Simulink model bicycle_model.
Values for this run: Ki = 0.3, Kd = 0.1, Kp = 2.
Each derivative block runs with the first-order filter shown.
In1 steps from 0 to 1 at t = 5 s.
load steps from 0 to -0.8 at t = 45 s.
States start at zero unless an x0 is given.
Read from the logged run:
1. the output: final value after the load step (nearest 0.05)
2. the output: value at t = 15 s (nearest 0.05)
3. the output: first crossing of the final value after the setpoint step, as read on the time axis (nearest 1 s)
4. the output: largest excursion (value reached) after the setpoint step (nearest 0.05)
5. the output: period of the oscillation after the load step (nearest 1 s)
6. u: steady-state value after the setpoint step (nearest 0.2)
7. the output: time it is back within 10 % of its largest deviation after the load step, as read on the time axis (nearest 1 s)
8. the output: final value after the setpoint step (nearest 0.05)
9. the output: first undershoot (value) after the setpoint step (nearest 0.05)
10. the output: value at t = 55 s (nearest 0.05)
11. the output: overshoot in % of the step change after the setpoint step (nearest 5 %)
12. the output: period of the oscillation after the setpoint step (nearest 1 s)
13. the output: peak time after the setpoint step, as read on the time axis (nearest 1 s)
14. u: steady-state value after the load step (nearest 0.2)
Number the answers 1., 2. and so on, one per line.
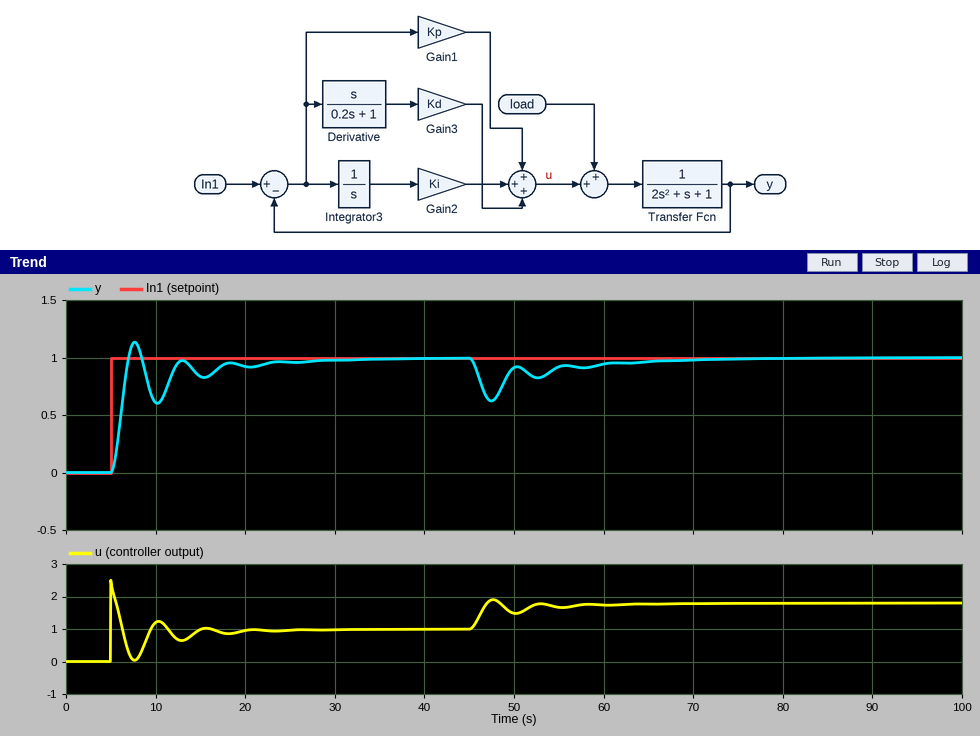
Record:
1. 1.00
2. 0.85
3. 7 s
4. 1.15
5. 5 s
6. 1.0
7. 65 s
8. 1.00
9. 0.60
10. 0.90
11. 15 %
12. 5 s
13. 8 s
14. 1.8
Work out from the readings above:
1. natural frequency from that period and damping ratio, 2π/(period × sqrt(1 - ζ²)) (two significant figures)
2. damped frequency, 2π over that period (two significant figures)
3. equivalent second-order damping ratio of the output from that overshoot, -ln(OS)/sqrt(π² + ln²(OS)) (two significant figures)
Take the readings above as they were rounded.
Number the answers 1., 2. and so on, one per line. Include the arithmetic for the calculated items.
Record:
1. 2π / (5 × sqrt(1 - 0.52²)) = 1.5 rad/s
2. 2π / 5 = 1.3 rad/s
3. ln(0.15) = -1.897; 1.897 / sqrt(9.870 + 3.599) = 0.52
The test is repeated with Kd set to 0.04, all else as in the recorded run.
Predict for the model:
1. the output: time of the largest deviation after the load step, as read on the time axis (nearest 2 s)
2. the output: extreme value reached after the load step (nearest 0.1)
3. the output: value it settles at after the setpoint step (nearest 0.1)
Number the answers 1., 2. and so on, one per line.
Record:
1. 48 s
2. 0.6
3. 1.0
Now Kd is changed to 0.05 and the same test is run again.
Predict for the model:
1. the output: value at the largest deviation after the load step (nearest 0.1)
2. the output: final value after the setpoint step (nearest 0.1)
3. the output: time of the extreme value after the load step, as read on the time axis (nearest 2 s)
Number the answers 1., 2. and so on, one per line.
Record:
1. 0.6
2. 1.0
3. 48 s
